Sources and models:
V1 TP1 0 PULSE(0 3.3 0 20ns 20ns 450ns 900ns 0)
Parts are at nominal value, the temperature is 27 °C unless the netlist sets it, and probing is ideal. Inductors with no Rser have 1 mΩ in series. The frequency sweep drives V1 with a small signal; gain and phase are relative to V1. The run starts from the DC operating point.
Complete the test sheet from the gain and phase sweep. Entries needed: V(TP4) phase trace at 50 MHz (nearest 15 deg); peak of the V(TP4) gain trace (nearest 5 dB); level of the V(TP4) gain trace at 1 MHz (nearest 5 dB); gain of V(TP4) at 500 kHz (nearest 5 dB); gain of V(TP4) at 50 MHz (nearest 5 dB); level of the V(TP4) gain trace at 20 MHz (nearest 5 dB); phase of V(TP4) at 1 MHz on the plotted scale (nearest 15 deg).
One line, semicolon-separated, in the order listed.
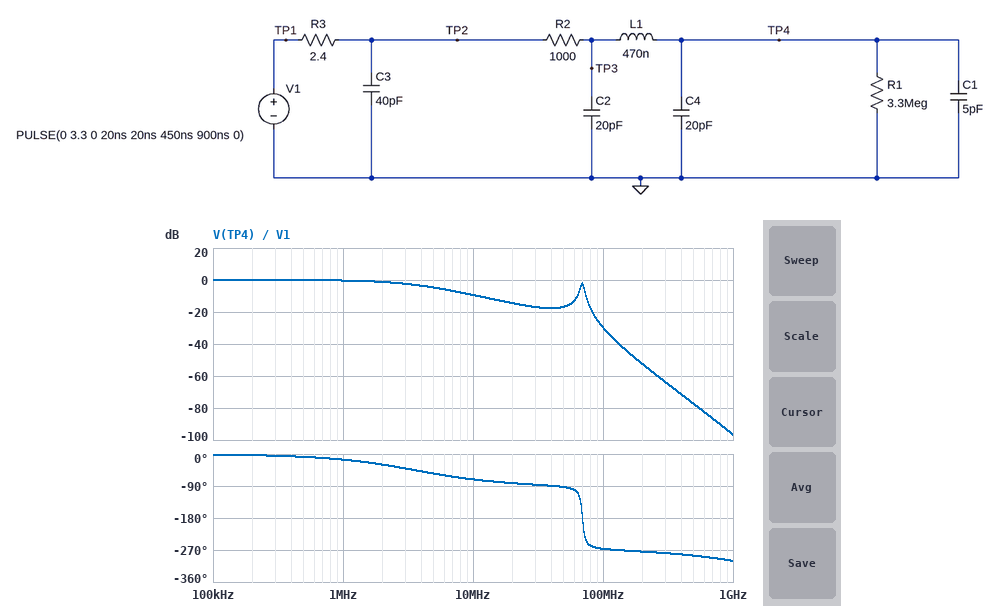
-90 deg; 0 dB; 0 dB; 0 dB; -15 dB; -15 dB; -15 deg
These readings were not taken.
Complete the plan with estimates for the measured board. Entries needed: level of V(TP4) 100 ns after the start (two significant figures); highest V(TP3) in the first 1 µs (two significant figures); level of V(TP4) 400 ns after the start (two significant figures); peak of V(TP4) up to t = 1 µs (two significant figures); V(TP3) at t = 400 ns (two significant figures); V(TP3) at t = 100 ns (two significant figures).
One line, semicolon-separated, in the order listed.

2.9 V; 3.3 V; 3.3 V; 3.3 V; 3.3 V; 2.8 V
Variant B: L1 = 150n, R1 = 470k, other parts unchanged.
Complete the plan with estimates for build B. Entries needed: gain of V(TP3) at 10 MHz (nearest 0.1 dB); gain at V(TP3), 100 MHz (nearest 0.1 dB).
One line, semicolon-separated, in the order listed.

-9.6 dB; -26.1 dB
